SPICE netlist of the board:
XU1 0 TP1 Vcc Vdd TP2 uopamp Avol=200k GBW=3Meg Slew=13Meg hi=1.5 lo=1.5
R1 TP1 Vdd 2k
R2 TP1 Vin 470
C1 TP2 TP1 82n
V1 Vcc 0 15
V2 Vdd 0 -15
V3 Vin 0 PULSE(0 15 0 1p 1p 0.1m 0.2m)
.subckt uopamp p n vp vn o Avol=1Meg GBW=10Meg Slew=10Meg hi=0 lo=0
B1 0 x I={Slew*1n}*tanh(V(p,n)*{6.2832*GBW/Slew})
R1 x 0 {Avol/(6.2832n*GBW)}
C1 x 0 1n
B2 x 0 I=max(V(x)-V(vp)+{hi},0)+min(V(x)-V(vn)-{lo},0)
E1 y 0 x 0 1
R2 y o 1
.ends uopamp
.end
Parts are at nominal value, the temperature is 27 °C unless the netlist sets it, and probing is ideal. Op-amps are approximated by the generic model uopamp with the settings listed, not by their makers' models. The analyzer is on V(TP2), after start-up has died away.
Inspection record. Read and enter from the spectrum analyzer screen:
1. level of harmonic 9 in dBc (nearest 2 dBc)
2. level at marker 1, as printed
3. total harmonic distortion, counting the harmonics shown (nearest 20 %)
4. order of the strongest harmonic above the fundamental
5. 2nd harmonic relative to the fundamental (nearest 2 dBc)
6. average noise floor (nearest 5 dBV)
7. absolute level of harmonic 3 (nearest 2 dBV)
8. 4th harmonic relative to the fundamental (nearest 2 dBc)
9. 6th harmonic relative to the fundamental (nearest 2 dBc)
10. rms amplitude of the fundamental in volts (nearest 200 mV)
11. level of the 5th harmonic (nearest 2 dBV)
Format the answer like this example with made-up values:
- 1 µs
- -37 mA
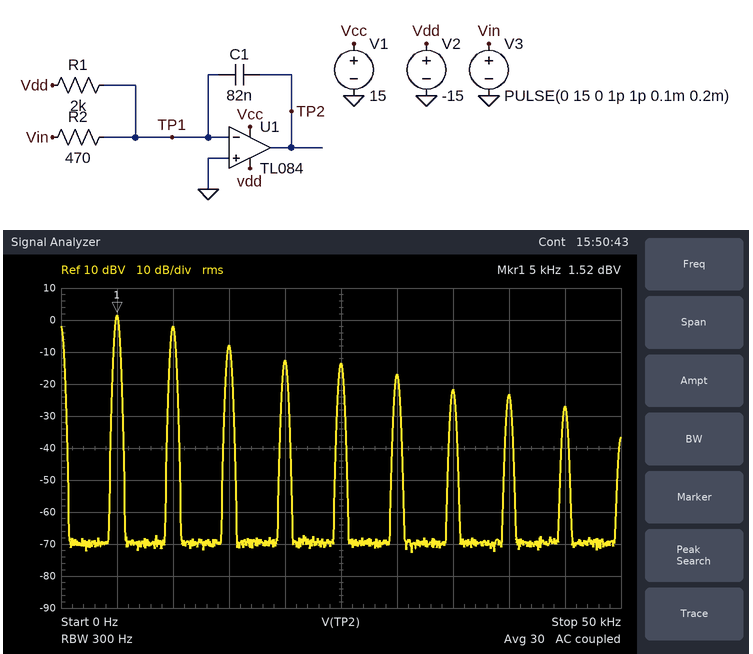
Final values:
- -28 dBc
- 1.52 dBV
- 80 %
- 2
- -4 dBc
- -70 dBV
- -8 dBV
- -14 dBc
- -18 dBc
- 1.2 V
- -14 dBV
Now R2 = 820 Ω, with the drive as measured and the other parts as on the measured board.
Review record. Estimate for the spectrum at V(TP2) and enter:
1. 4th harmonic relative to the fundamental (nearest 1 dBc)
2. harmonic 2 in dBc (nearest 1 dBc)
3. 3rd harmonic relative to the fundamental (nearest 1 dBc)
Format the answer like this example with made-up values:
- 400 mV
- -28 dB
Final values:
- -27 dBc
- -8 dBc
- -21 dBc
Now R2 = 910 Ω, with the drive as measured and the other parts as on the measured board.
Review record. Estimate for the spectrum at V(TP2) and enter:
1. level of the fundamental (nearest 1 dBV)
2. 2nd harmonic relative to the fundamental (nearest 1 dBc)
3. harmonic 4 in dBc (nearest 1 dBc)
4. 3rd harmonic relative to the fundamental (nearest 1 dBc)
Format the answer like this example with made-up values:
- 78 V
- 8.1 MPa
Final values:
- 7 dBV
- -13 dBc
- -24 dBc
- -28 dBc
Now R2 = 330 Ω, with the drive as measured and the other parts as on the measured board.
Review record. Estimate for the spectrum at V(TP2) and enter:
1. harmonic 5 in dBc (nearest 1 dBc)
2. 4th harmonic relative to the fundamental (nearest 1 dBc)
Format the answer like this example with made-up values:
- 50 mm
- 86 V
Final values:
- -14 dBc
- -13 dBc
